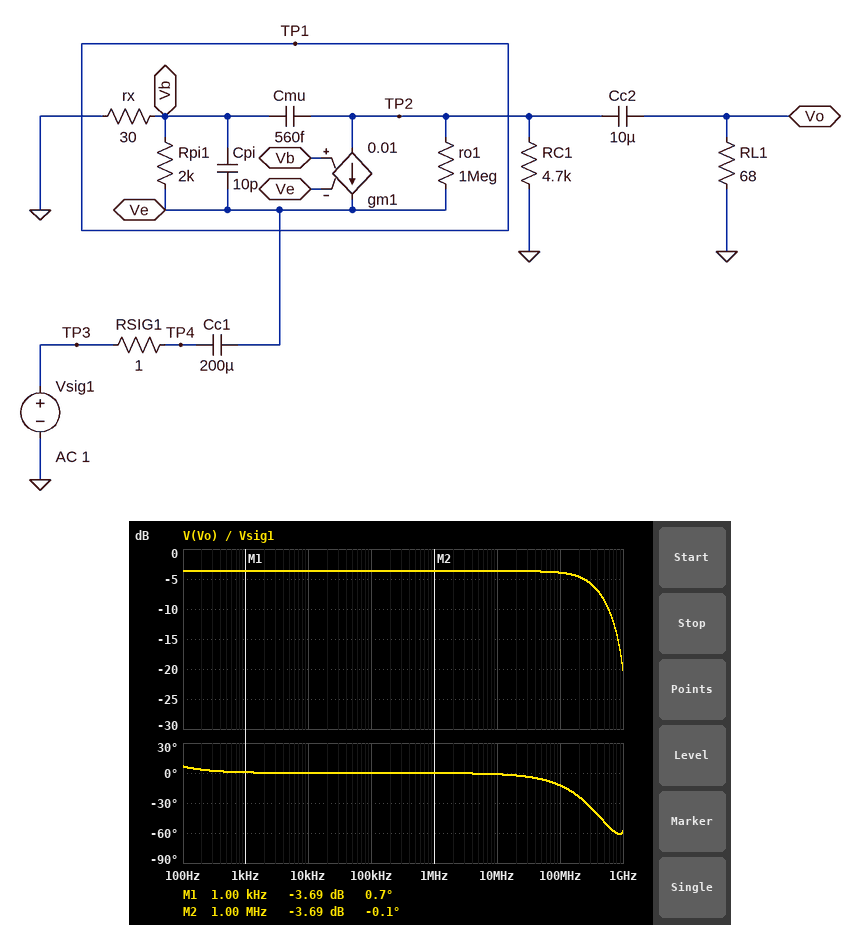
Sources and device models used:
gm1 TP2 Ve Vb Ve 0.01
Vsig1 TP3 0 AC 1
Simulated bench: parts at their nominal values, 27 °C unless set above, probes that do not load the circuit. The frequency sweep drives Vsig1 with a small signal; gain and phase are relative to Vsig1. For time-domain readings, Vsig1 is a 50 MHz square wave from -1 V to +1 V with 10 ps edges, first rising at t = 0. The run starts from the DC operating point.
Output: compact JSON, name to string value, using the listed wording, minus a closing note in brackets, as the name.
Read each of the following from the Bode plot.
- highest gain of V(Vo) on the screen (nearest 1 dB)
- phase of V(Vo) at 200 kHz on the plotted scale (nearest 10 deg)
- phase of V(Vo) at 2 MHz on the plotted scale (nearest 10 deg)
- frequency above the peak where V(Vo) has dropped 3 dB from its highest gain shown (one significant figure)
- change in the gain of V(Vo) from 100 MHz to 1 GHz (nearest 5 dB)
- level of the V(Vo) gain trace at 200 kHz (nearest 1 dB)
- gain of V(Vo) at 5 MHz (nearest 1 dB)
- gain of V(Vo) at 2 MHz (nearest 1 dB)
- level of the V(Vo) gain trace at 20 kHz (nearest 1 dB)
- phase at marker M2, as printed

{"highest gain of V(Vo) on the screen": "-4 dB", "phase of V(Vo) at 200 kHz on the plotted scale": "0 deg", "phase of V(Vo) at 2 MHz on the plotted scale": "0 deg", "frequency above the peak where V(Vo) has dropped 3 dB from its highest gain shown": "400 MHz", "change in the gain of V(Vo) from 100 MHz to 1 GHz": "-15 dB", "level of the V(Vo) gain trace at 200 kHz": "-4 dB", "gain of V(Vo) at 5 MHz": "-4 dB", "gain of V(Vo) at 2 MHz": "-4 dB", "level of the V(Vo) gain trace at 20 kHz": "-4 dB", "phase at marker M2, as printed": "-0.1 deg"}
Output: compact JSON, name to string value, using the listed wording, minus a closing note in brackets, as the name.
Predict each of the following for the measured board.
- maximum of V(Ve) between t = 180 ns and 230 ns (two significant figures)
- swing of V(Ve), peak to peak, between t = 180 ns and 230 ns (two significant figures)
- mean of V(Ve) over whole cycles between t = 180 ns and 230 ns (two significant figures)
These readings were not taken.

{"maximum of V(Ve) between t = 180 ns and 230 ns": "2.0 V", "swing of V(Ve), peak to peak, between t = 180 ns and 230 ns": "2.0 V", "mean of V(Ve) over whole cycles between t = 180 ns and 230 ns": "990 mV"}
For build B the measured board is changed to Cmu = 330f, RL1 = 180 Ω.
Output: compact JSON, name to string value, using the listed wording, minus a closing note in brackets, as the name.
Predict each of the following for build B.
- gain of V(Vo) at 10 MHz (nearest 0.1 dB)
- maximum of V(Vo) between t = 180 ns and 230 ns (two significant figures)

{"gain of V(Vo) at 10 MHz": "4.6 dB", "maximum of V(Vo) between t = 180 ns and 230 ns": "3.4 V"}
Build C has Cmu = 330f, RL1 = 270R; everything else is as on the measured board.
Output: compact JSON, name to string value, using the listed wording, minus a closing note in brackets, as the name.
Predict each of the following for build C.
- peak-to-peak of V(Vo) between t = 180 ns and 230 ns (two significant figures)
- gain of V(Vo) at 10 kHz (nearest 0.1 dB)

{"peak-to-peak of V(Vo) between t = 180 ns and 230 ns": "5.0 V", "gain of V(Vo) at 10 kHz": "7.9 dB"}
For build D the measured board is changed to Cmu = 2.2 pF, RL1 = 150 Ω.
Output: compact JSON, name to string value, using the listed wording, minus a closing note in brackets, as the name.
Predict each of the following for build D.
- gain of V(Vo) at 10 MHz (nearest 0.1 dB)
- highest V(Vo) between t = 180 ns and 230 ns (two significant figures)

{"gain of V(Vo) at 10 MHz": "3.0 dB", "highest V(Vo) between t = 180 ns and 230 ns": "2.8 V"}
